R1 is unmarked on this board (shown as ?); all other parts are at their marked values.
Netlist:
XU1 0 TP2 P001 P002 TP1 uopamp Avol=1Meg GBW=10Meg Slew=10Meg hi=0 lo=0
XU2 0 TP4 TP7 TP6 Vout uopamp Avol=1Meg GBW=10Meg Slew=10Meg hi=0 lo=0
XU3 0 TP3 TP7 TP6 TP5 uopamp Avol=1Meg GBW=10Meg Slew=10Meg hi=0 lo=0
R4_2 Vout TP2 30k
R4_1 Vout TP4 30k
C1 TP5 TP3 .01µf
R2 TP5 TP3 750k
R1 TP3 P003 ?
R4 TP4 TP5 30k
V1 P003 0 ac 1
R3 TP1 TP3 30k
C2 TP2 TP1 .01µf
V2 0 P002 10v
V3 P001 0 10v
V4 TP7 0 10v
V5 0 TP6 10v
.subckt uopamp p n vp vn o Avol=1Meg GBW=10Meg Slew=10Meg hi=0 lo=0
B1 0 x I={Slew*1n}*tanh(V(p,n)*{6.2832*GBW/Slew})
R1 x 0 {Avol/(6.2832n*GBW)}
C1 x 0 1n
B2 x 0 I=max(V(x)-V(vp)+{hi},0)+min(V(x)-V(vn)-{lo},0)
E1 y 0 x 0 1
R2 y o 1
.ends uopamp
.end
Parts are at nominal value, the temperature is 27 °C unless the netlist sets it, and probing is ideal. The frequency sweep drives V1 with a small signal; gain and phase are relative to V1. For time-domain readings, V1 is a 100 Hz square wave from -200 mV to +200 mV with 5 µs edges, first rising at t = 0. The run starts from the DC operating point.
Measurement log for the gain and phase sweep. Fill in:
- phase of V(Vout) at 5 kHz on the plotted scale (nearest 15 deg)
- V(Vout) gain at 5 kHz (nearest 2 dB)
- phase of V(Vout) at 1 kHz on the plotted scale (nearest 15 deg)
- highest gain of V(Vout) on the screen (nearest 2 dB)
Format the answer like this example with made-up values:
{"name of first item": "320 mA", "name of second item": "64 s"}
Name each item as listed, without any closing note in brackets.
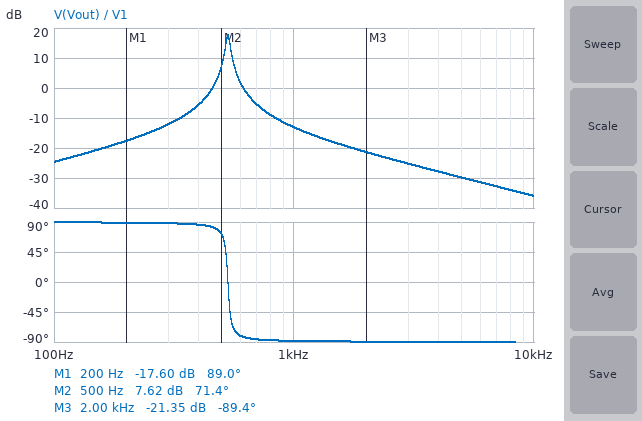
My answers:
{"phase of V(Vout) at 5 kHz on the plotted scale": "-90 deg", "V(Vout) gain at 5 kHz": "-30 dB", "phase of V(Vout) at 1 kHz on the plotted scale": "-90 deg", "highest gain of V(Vout) on the screen": "18 dB"}
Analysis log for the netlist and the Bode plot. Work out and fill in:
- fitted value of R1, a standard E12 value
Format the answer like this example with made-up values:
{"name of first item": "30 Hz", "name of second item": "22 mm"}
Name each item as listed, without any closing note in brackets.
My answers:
{"fitted value of R1, a standard E12 value": "100 kΩ"}
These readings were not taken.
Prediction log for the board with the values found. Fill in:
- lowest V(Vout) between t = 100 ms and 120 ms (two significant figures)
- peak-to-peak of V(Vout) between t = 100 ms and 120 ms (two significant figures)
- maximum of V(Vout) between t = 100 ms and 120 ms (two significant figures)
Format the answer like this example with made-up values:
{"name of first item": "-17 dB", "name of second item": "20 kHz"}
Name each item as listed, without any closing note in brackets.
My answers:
{"lowest V(Vout) between t = 100 ms and 120 ms": "-140 mV", "peak-to-peak of V(Vout) between t = 100 ms and 120 ms": "290 mV", "maximum of V(Vout) between t = 100 ms and 120 ms": "140 mV"}
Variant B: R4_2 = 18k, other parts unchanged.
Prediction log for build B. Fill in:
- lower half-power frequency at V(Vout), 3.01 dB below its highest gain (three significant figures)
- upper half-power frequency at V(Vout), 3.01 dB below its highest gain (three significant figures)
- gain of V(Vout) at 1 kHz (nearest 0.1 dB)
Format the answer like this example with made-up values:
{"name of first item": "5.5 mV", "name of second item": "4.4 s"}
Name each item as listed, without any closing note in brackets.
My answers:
{"lower half-power frequency at V(Vout), 3.01 dB below its highest gain": "674 Hz", "upper half-power frequency at V(Vout), 3.01 dB below its highest gain": "695 Hz", "gain of V(Vout) at 1 kHz": "-10.5 dB"}
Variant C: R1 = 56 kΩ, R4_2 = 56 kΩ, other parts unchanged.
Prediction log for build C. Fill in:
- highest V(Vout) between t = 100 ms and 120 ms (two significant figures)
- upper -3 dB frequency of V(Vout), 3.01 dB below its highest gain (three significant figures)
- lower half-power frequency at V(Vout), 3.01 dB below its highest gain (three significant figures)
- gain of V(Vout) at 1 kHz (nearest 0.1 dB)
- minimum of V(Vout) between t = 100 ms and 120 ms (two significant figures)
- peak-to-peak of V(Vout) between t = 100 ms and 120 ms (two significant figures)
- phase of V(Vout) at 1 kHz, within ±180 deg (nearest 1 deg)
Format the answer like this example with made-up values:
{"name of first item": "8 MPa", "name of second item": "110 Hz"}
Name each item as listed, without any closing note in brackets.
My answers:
{"highest V(Vout) between t = 100 ms and 120 ms": "170 mV", "upper -3 dB frequency of V(Vout), 3.01 dB below its highest gain": "399 Hz", "lower half-power frequency at V(Vout), 3.01 dB below its highest gain": "378 Hz", "gain of V(Vout) at 1 kHz": "-9.5 dB", "minimum of V(Vout) between t = 100 ms and 120 ms": "-170 mV", "peak-to-peak of V(Vout) between t = 100 ms and 120 ms": "330 mV", "phase of V(Vout) at 1 kHz, within ±180 deg": "-89 deg"}
